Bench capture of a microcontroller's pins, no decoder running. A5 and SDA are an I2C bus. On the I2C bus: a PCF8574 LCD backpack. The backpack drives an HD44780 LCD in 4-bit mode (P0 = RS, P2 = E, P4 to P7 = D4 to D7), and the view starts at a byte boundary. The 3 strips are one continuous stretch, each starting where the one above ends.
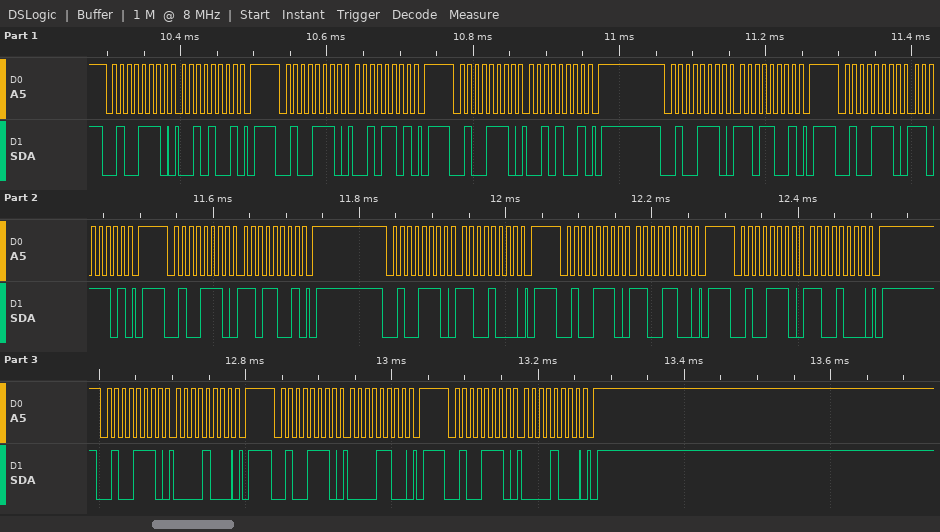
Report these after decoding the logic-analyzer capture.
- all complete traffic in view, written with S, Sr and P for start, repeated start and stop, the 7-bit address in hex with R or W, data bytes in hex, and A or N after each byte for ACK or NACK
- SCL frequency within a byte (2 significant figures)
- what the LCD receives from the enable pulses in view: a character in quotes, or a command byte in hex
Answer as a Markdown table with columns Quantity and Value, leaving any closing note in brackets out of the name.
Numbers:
| Quantity | Value |
|---|---|
| all complete traffic in view, written with S, Sr and P for start, repeated start and stop, the 7-bit address in hex with R or W, data bytes in hex, and A or N after each byte for ACK or NACK | S 27W A 29 A P S 27W A 2D A P S 27W A 29 A P S 27W A D9 A P S 27W A DD A P S 27W A D9 A P S 27W A C8 A P S 27W A CC A P S 27W A C8 A P S 27W A 08 A P S 27W A 0C A P S 27W A 08 A P |
| SCL frequency within a byte | 100 kHz |
| what the LCD receives from the enable pulses in view: a character in quotes, or a command byte in hex | '-' 0xC0 |
